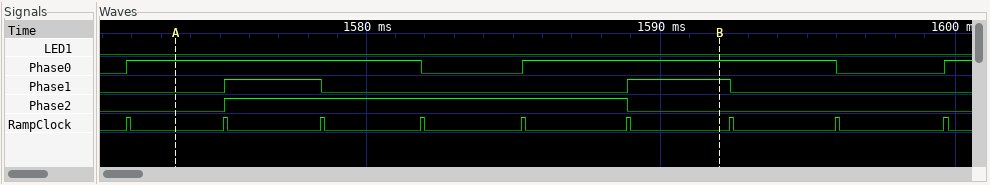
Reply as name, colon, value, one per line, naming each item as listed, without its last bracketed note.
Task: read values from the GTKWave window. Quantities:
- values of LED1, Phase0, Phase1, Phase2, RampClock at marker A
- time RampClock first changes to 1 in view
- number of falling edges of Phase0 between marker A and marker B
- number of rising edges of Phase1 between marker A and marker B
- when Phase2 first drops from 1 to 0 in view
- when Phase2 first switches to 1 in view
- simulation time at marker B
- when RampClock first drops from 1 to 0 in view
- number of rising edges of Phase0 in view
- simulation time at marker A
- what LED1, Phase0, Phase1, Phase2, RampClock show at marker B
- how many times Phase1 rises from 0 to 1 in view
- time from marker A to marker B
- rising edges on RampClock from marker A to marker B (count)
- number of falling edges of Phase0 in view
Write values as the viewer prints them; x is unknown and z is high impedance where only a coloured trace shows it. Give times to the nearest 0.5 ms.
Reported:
values of LED1, Phase0, Phase1, Phase2, RampClock at marker A: LED1=0, Phase0=1, Phase1=0, Phase2=0, RampClock=0
time RampClock first changes to 1 in view: 1572 ms
number of falling edges of Phase0 between marker A and marker B: 1
number of rising edges of Phase1 between marker A and marker B: 2
when Phase2 first drops from 1 to 0 in view: 1589 ms
when Phase2 first switches to 1 in view: 1575 ms
simulation time at marker B: 1592 ms
when RampClock first drops from 1 to 0 in view: 1572 ms
number of rising edges of Phase0 in view: 3
simulation time at marker A: 1573.5 ms
what LED1, Phase0, Phase1, Phase2, RampClock show at marker B: LED1=0, Phase0=1, Phase1=1, Phase2=0, RampClock=0
how many times Phase1 rises from 0 to 1 in view: 2
time from marker A to marker B: 18.5 ms
rising edges on RampClock from marker A to marker B: 5
number of falling edges of Phase0 in view: 2
